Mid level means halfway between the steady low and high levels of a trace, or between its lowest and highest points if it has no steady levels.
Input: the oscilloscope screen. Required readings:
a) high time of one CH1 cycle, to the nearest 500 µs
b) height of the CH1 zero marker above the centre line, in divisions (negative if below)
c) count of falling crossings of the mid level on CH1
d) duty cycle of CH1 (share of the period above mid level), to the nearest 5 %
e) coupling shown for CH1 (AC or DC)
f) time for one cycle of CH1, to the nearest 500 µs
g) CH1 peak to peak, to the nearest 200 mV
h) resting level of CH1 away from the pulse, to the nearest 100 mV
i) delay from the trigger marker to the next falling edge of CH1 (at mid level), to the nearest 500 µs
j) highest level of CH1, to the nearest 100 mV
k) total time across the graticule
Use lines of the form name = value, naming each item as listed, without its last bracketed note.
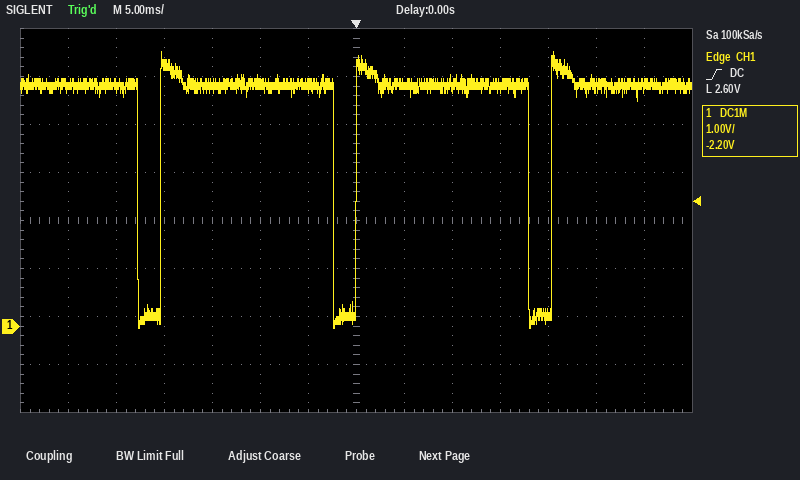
high time of one CH1 cycle, to the nearest 500 µs = 18.0 ms
height of the CH1 zero marker above the centre line, in divisions = -2.2 div
count of falling crossings of the mid level on CH1 = 3
duty cycle of CH1 (share of the period above mid level), to the nearest 5 % = 90 %
coupling shown for CH1 = DC
time for one cycle of CH1, to the nearest 500 µs = 20.5 ms
CH1 peak to peak, to the nearest 200 mV = 5.8 V
resting level of CH1 away from the pulse, to the nearest 100 mV = 5.0 V
delay from the trigger marker to the next falling edge of CH1 (at mid level), to the nearest 500 µs = 18.0 ms
highest level of CH1, to the nearest 100 mV = 5.7 V
total time across the graticule = 70 ms
